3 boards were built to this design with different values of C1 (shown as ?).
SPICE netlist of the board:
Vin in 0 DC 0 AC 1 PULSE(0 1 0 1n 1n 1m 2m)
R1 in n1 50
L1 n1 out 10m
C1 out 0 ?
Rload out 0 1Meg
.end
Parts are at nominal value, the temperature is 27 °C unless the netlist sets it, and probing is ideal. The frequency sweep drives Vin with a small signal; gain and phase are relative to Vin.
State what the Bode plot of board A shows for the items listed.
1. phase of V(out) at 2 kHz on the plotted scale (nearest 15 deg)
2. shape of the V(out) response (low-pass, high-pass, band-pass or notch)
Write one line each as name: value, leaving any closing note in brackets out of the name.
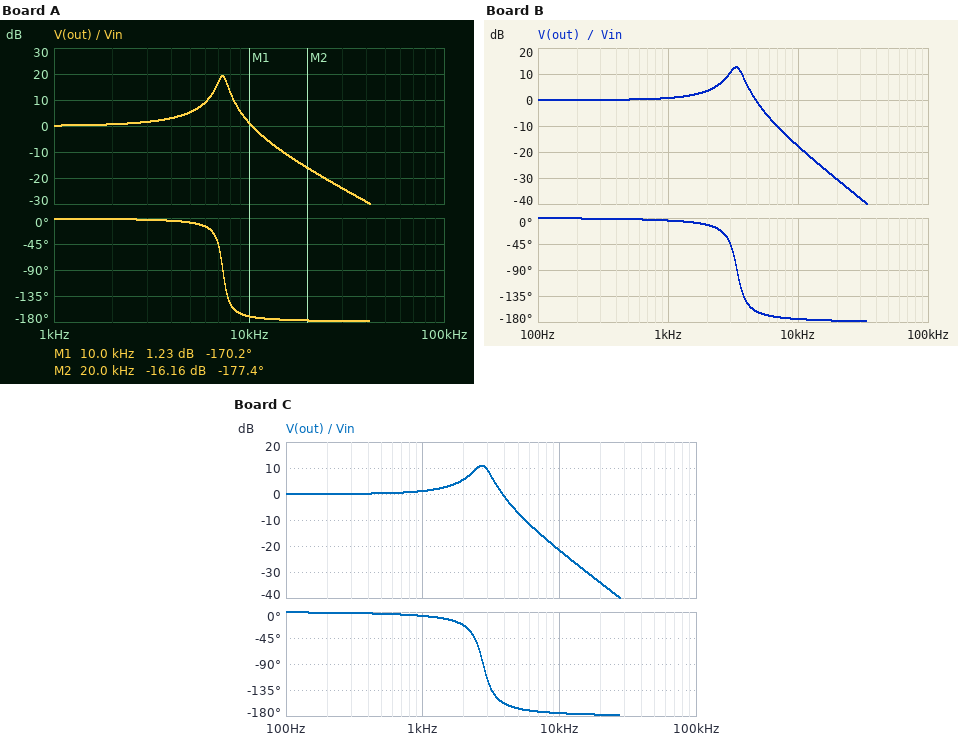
phase of V(out) at 2 kHz on the plotted scale: 0 deg
shape of the V(out) response: low-pass
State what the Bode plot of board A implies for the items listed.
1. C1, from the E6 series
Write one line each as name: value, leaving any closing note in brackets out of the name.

C1, from the E6 series: 47 nF
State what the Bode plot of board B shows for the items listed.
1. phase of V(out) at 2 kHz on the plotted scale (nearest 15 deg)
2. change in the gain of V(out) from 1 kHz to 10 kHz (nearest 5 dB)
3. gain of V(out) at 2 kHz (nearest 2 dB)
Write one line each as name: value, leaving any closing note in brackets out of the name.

phase of V(out) at 2 kHz on the plotted scale: -15 deg
change in the gain of V(out) from 1 kHz to 10 kHz: -20 dB
gain of V(out) at 2 kHz: 4 dB
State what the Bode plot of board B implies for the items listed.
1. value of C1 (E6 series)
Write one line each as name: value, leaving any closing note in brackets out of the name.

value of C1: 220 nF
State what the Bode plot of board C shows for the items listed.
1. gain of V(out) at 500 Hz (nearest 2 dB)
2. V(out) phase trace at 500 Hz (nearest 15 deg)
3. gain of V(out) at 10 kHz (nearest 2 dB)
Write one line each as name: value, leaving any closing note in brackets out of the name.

gain of V(out) at 500 Hz: 0 dB
V(out) phase trace at 500 Hz: 0 deg
gain of V(out) at 10 kHz: -22 dB
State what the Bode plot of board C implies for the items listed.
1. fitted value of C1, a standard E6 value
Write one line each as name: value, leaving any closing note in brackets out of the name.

fitted value of C1, a standard E6 value: 330 nF
